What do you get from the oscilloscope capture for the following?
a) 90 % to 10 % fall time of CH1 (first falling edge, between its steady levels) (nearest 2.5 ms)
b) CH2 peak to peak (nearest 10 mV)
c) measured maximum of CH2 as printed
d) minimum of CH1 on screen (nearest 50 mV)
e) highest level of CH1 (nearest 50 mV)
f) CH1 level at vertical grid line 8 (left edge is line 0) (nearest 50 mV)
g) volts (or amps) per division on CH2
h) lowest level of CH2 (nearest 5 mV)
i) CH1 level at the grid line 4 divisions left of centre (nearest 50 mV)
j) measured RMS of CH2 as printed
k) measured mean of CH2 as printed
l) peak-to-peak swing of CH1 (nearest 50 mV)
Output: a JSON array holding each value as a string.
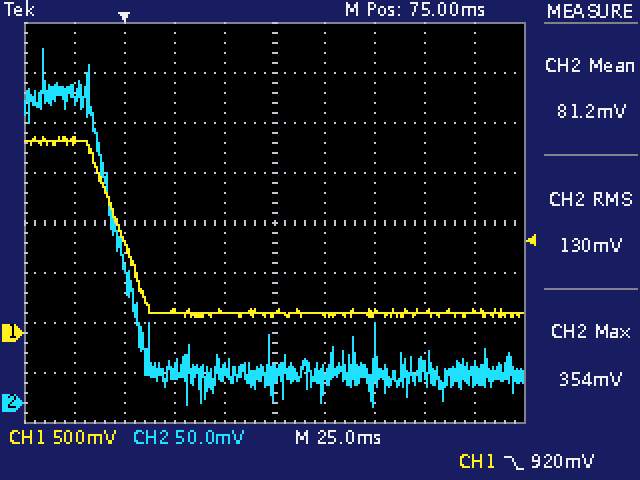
["25.0 ms", "360 mV", "354 mV", "150 mV", "1.95 V", "200 mV", "50 mV", "-5 mV", "1.90 V", "130 mV", "81.2 mV", "1.80 V"]
